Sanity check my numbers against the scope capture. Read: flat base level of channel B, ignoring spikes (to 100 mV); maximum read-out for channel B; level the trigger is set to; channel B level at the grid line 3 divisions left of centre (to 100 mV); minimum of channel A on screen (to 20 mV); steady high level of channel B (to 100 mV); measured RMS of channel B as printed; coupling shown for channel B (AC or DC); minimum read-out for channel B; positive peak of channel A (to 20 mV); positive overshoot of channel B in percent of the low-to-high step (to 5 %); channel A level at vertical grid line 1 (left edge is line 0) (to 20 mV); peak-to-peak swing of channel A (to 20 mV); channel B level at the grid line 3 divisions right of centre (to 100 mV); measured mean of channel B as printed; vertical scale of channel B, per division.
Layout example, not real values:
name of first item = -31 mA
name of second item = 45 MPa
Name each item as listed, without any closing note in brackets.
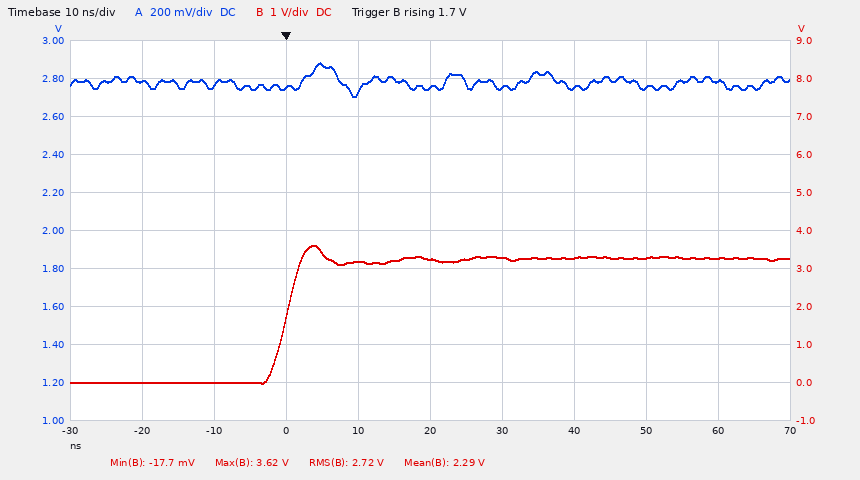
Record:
flat base level of channel B, ignoring spikes = 0.0 V
maximum read-out for channel B = 3.62 V
level the trigger is set to = 1.7 V
channel B level at the grid line 3 divisions left of centre = 0.0 V
minimum of channel A on screen = 2.70 V
steady high level of channel B = 3.3 V
measured RMS of channel B as printed = 2.72 V
coupling shown for channel B = DC
minimum read-out for channel B = -17.7 mV
positive peak of channel A = 2.88 V
positive overshoot of channel B in percent of the low-to-high step = 10 %
channel A level at vertical grid line 1 (left edge is line 0) = 2.78 V
peak-to-peak swing of channel A = 180 mV
channel B level at the grid line 3 divisions right of centre = 3.3 V
measured mean of channel B as printed = 2.29 V
vertical scale of channel B, per division = 1 V
